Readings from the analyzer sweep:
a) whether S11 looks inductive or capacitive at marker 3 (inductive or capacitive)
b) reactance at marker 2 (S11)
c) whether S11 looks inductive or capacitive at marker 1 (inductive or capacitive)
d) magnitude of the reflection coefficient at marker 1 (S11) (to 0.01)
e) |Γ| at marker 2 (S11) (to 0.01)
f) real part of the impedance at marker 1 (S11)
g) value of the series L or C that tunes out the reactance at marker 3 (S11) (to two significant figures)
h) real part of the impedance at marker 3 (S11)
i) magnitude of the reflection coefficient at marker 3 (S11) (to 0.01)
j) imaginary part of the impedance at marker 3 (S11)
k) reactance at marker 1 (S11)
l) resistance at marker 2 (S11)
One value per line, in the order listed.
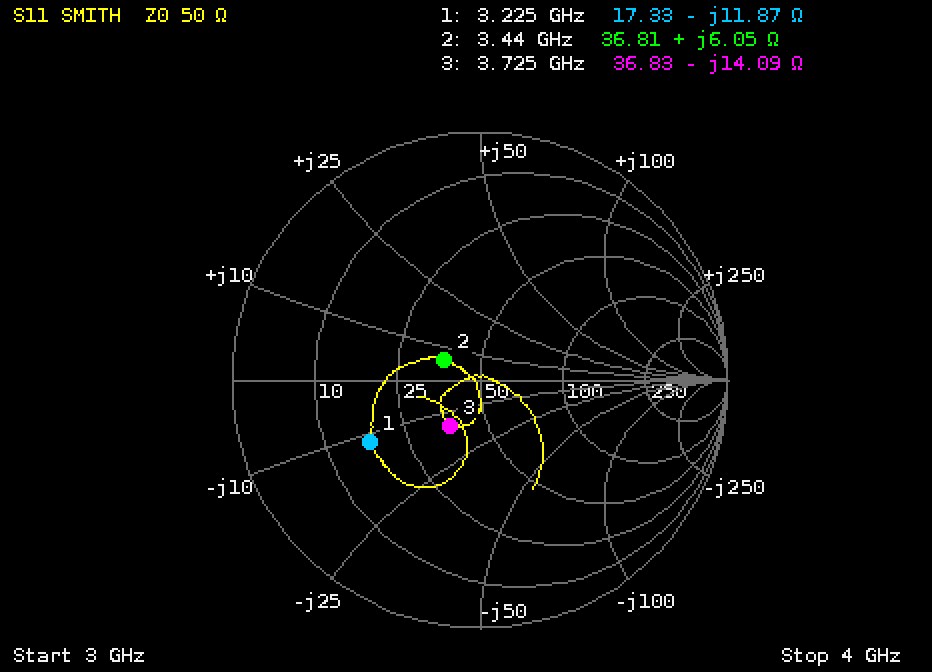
capacitive
+6.05 Ω
capacitive
0.51
0.17
17.33 Ω
600 pH
36.83 Ω
0.22
-14.09 Ω
-11.87 Ω
36.81 Ω
